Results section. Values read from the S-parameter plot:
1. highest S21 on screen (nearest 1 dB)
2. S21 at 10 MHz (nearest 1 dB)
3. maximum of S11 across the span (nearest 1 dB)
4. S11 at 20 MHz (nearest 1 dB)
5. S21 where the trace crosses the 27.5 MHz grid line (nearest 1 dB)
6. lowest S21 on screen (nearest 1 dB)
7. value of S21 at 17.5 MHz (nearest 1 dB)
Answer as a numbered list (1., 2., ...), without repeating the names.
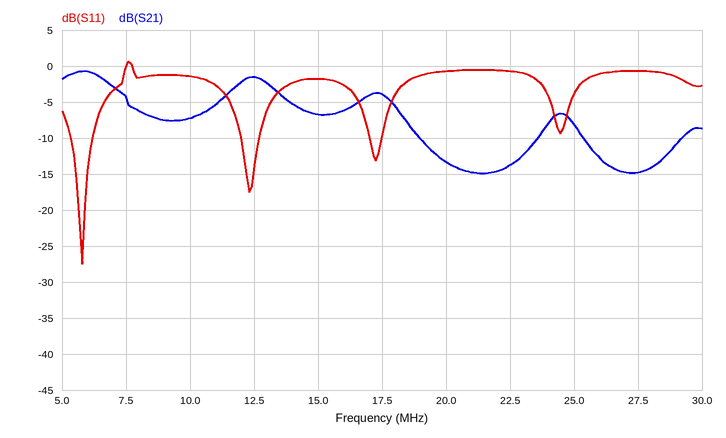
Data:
1. -1 dB
2. -7 dB
3. 1 dB
4. -1 dB
5. -15 dB
6. -15 dB
7. -4 dB
